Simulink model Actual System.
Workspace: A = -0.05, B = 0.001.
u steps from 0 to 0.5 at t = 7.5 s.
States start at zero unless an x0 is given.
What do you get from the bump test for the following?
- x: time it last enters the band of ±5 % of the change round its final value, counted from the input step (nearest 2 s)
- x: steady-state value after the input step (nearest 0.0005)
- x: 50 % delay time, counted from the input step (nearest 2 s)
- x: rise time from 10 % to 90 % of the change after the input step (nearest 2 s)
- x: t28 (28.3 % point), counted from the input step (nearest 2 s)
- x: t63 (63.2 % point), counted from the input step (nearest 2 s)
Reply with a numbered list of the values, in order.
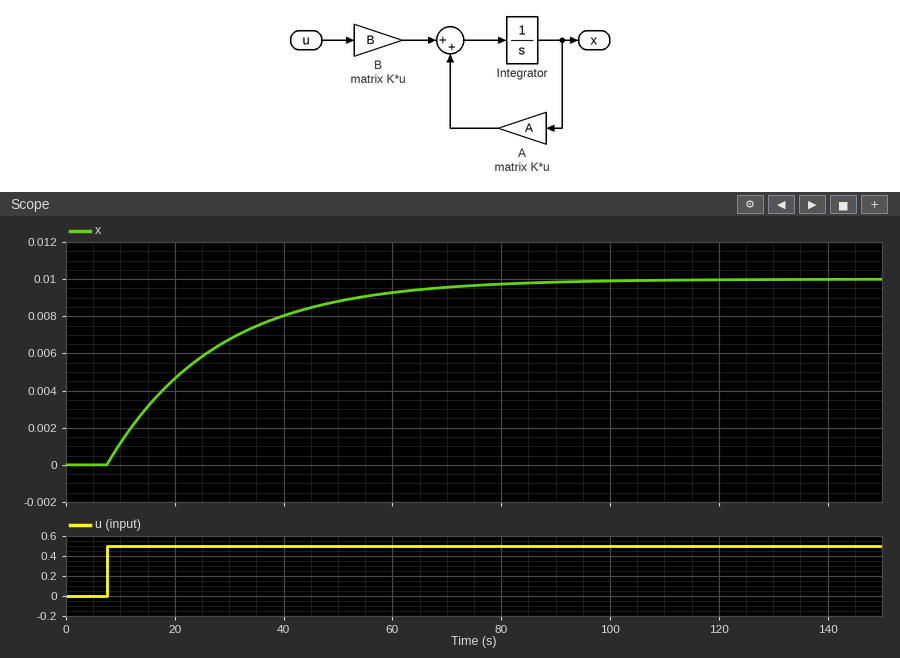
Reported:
1. 60 s
2. 0.0100
3. 14 s
4. 44 s
5. 6 s
6. 20 s
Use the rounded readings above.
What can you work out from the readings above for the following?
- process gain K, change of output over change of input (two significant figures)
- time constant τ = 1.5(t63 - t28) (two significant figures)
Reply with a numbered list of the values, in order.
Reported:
1. 0.020
2. 21 s
